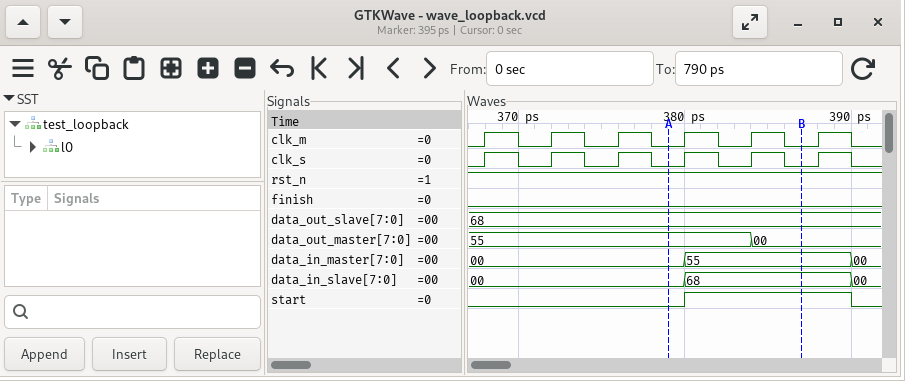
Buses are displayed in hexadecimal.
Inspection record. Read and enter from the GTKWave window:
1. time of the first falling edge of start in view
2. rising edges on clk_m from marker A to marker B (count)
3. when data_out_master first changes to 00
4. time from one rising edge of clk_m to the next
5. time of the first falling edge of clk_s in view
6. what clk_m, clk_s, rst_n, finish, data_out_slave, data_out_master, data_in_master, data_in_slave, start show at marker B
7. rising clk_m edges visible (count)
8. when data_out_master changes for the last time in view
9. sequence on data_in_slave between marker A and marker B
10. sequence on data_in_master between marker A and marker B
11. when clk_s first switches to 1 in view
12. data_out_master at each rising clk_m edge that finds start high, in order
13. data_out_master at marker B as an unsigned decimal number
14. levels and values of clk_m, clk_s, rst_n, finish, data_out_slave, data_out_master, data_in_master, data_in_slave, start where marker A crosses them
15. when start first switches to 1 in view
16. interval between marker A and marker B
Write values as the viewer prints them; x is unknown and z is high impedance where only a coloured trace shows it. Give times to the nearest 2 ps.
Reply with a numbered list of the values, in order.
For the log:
1. 390 ps
2. 2
3. 384 ps
4. 4 ps
5. 370 ps
6. clk_m=0, clk_s=0, rst_n=1, finish=0, data_out_slave=68, data_out_master=00, data_in_master=55, data_in_slave=68, start=1
7. 6
8. 384 ps
9. 00, 68
10. 00, 55
11. 368 ps
12. 55, 00
13. 0
14. clk_m=0, clk_s=0, rst_n=1, finish=0, data_out_slave=68, data_out_master=55, data_in_master=00, data_in_slave=00, start=0
15. 380 ps
16. 8 ps
